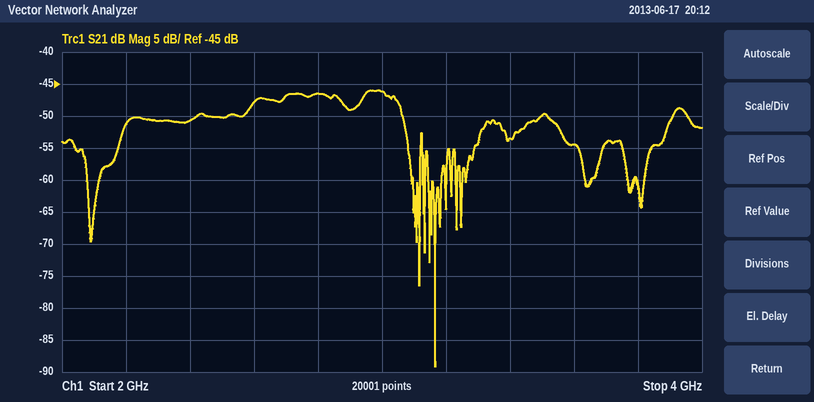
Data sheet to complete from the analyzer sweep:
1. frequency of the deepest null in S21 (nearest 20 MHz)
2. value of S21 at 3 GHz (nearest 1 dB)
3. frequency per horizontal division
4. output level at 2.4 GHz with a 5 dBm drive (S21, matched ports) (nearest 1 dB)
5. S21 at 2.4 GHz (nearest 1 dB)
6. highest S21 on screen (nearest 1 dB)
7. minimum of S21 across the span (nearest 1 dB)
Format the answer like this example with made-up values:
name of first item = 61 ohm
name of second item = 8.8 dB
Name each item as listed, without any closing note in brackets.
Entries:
frequency of the deepest null in S21 = 3.16 GHz
value of S21 at 3 GHz = -46 dB
frequency per horizontal division = 200 MHz
output level at 2.4 GHz with a 5 dBm drive (S21, matched ports) = -46 dBm
S21 at 2.4 GHz = -51 dB
highest S21 on screen = -46 dB
minimum of S21 across the span = -89 dB
